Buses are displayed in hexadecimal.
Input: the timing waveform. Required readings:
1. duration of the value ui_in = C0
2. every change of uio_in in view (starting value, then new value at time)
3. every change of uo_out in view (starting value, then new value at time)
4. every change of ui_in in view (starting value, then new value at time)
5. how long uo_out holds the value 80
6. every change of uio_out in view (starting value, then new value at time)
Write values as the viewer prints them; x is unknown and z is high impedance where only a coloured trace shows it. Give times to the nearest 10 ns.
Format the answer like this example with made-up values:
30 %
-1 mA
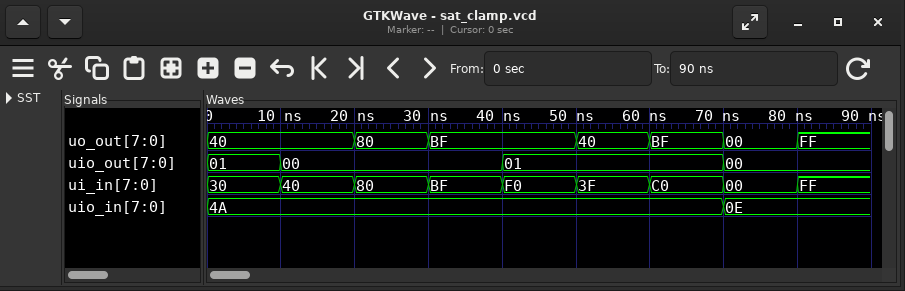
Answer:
10 ns
4A, 0E at 70 ns
40, 80 at 20 ns, BF at 30 ns, 40 at 50 ns, BF at 60 ns, 00 at 70 ns, FF at 80 ns
30, 40 at 10 ns, 80 at 20 ns, BF at 30 ns, F0 at 40 ns, 3F at 50 ns, C0 at 60 ns, 00 at 70 ns, FF at 80 ns
10 ns
01, 00 at 10 ns, 01 at 40 ns, 00 at 70 ns
